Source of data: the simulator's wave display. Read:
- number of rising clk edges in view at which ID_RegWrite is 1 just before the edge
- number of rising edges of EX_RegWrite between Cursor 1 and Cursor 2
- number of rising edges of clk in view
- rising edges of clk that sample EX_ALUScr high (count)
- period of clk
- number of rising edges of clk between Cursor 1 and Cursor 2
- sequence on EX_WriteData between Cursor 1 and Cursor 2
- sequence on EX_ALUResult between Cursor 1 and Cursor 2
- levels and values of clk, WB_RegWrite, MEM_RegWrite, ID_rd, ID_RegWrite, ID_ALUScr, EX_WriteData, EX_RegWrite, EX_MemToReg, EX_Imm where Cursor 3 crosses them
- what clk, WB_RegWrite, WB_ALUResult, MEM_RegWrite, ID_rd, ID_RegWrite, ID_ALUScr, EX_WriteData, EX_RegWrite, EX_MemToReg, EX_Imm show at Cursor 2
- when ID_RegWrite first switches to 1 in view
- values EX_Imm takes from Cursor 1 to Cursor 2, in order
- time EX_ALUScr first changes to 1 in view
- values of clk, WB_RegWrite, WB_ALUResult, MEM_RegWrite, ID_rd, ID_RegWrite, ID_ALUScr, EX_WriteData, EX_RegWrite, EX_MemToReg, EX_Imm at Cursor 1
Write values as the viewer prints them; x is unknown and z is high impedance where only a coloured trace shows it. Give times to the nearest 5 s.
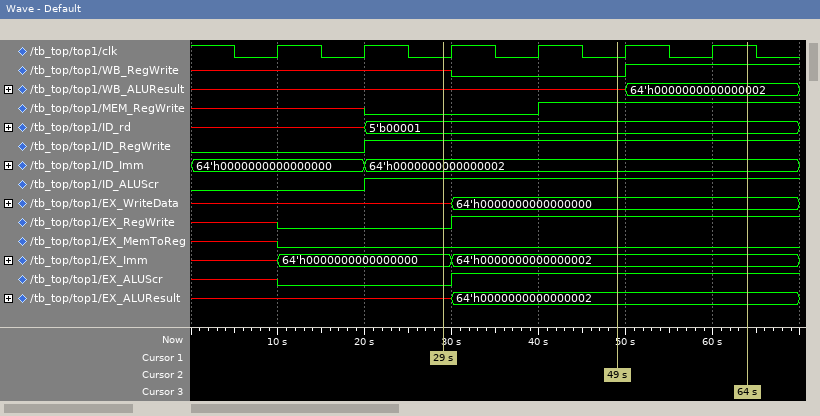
4
1
6
3
10 s
2
x, 64'h0000000000000000
x, 64'h0000000000000002
clk=1, WB_RegWrite=1, MEM_RegWrite=1, ID_rd=5'b00001, ID_RegWrite=1, ID_ALUScr=1, EX_WriteData=64'h0000000000000000, EX_RegWrite=1, EX_MemToReg=0, EX_Imm=64'h0000000000000002
clk=0, WB_RegWrite=0, WB_ALUResult=x, MEM_RegWrite=1, ID_rd=5'b00001, ID_RegWrite=1, ID_ALUScr=1, EX_WriteData=64'h0000000000000000, EX_RegWrite=1, EX_MemToReg=0, EX_Imm=64'h0000000000000002
20 s
64'h0000000000000000, 64'h0000000000000002
30 s
clk=0, WB_RegWrite=x, WB_ALUResult=x, MEM_RegWrite=0, ID_rd=5'b00001, ID_RegWrite=1, ID_ALUScr=1, EX_WriteData=x, EX_RegWrite=0, EX_MemToReg=0, EX_Imm=64'h0000000000000000
